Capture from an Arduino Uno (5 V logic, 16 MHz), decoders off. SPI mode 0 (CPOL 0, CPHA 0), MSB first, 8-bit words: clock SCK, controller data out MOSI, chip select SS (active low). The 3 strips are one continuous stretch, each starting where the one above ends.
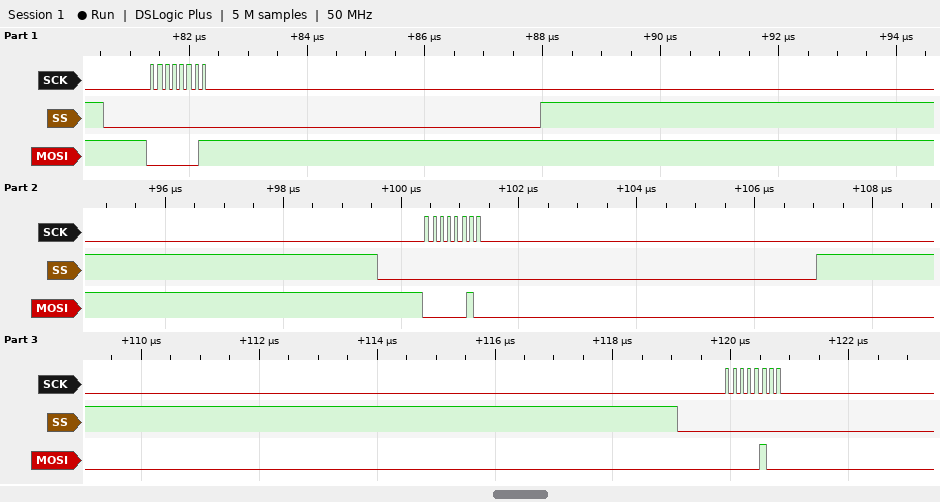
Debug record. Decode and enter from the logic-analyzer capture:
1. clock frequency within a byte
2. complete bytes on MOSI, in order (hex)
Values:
8 MHz
0x01 0x02 0x04
